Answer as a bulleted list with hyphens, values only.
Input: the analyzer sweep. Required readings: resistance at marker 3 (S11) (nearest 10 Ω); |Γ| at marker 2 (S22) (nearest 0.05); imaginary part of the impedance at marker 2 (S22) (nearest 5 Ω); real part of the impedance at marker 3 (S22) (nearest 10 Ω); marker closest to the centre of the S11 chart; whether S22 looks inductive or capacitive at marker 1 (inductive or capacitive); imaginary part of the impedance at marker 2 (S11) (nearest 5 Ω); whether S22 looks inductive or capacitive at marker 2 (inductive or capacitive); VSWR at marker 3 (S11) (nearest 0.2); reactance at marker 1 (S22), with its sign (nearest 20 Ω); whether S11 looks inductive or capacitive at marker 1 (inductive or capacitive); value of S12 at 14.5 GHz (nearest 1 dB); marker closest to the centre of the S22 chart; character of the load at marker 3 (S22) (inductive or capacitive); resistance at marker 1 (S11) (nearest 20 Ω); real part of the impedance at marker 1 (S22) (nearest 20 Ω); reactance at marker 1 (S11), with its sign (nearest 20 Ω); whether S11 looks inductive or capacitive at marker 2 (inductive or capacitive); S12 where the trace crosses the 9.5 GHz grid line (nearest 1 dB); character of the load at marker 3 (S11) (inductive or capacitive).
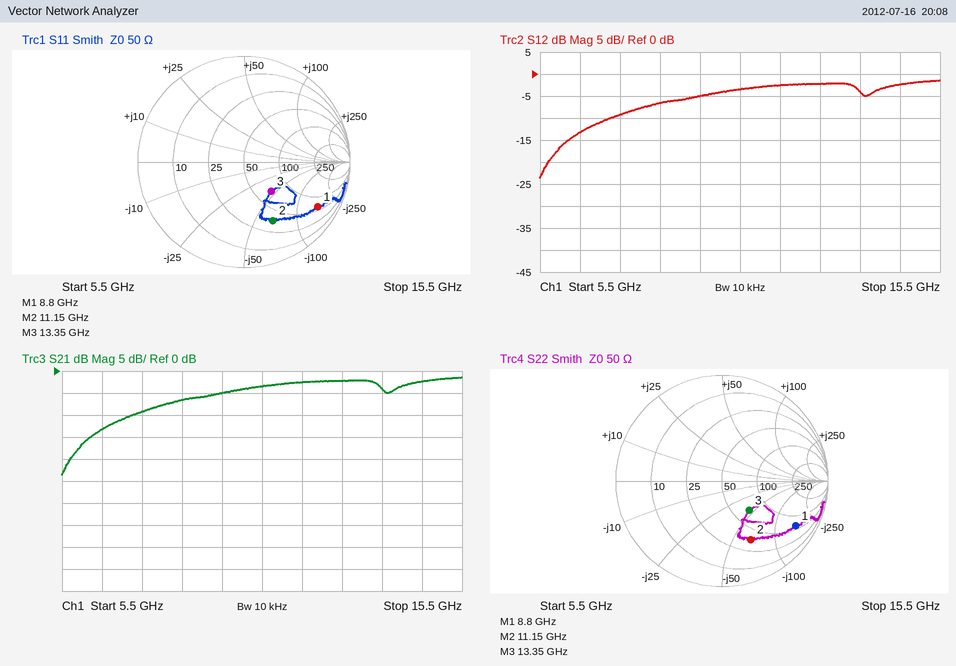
- 70 Ω
- 0.60
- -65 Ω
- 70 Ω
- marker 3
- capacitive
- -65 Ω
- capacitive
- 2.2
- -160 Ω
- capacitive
- -2 dB
- marker 3
- capacitive
- 60 Ω
- 60 Ω
- -160 Ω
- capacitive
- -5 dB
- capacitive
